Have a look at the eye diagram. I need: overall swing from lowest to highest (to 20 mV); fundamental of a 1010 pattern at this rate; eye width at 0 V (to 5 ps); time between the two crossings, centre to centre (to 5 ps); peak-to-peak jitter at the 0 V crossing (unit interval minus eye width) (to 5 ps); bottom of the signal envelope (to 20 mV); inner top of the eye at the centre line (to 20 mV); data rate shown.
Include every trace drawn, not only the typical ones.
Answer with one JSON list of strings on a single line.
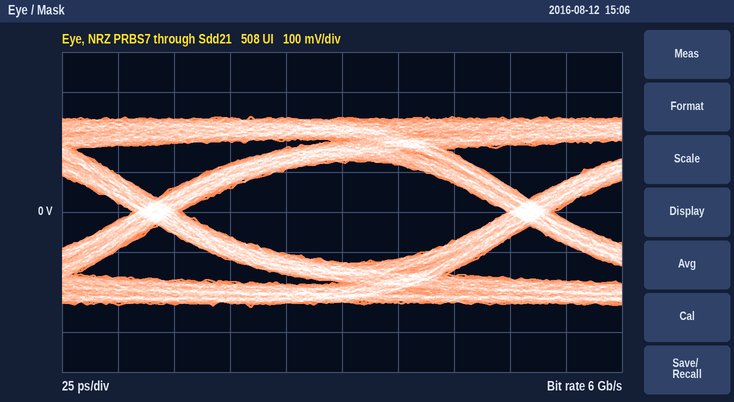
["480 mV", "3 GHz", "145 ps", "165 ps", "20 ps", "-240 mV", "120 mV", "6 Gb/s"]
